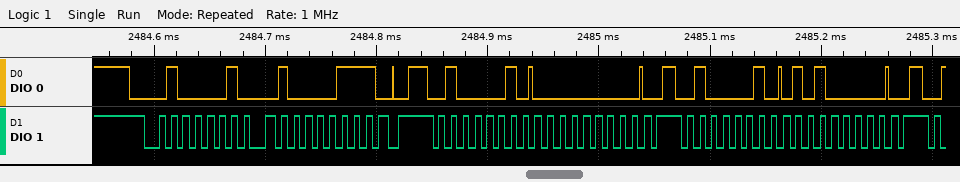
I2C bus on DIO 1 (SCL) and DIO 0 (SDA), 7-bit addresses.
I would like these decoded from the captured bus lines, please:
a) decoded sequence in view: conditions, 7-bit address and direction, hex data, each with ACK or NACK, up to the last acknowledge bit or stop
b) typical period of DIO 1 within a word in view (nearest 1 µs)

start, address 21 write ACK, 87 ACK, stop, start, address 21 write ACK, 00 ACK, stop, start, address 21 write ACK, A0 ACK, stop
11 µs
